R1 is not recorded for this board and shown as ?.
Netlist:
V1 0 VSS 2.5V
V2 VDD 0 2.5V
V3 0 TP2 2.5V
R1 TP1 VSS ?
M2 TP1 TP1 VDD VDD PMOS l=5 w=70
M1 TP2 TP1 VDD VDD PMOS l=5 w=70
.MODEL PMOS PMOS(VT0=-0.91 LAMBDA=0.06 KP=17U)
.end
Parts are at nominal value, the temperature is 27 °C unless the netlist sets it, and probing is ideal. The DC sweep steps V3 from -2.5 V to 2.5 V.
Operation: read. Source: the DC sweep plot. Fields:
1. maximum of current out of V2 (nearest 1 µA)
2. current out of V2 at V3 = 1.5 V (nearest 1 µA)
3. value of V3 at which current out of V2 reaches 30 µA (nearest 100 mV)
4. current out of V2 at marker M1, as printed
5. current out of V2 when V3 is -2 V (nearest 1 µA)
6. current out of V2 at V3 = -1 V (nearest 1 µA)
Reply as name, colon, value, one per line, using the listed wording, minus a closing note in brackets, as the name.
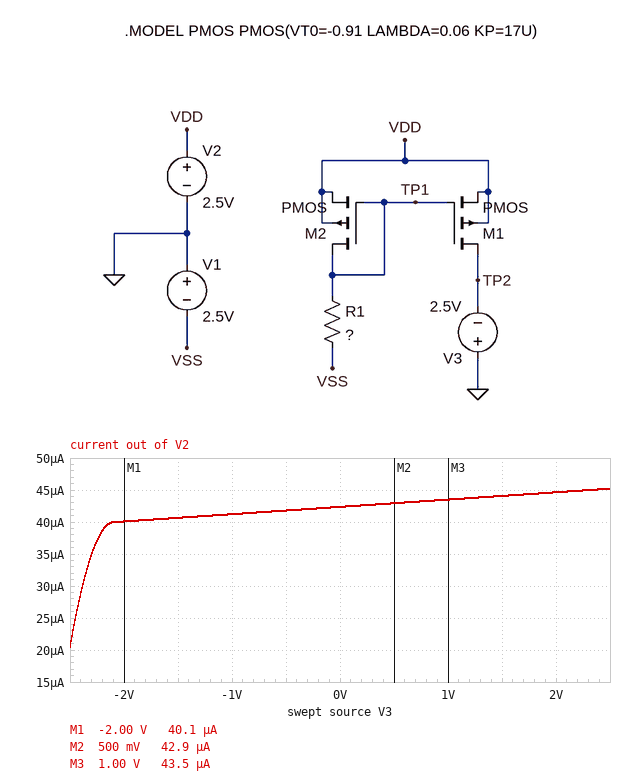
maximum of current out of V2: 45 µA
current out of V2 at V3 = 1.5 V: 44 µA
value of V3 at which current out of V2 reaches 30 µA: -2.4 V
current out of V2 at marker M1, as printed: 40.1 µA
current out of V2 when V3 is -2 V: 40 µA
current out of V2 at V3 = -1 V: 41 µA
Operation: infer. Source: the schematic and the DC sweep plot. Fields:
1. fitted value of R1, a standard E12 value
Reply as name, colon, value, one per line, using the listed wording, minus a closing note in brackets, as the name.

fitted value of R1, a standard E12 value: 180 kΩ
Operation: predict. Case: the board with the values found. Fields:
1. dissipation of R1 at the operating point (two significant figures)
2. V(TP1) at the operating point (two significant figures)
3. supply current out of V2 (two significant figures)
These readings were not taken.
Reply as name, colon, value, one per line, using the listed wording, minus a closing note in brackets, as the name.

dissipation of R1 at the operating point: 76 µW
V(TP1) at the operating point: 1.2 V
supply current out of V2: 45 µA
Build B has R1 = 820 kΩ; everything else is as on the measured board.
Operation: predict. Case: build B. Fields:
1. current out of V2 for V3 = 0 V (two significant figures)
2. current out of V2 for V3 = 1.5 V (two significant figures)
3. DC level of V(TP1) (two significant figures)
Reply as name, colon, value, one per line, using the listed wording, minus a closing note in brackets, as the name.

current out of V2 for V3 = 0 V: 9.9 µA
current out of V2 for V3 = 1.5 V: 10 µA
DC level of V(TP1): 1.4 V
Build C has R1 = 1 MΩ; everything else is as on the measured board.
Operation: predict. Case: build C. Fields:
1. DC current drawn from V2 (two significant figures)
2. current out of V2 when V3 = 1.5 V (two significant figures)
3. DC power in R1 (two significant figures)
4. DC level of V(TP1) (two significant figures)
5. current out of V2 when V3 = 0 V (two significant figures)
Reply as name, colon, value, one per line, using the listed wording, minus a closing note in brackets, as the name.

DC current drawn from V2: 8.7 µA
current out of V2 when V3 = 1.5 V: 8.5 µA
DC power in R1: 15 µW
DC level of V(TP1): 1.4 V
current out of V2 when V3 = 0 V: 8.1 µA
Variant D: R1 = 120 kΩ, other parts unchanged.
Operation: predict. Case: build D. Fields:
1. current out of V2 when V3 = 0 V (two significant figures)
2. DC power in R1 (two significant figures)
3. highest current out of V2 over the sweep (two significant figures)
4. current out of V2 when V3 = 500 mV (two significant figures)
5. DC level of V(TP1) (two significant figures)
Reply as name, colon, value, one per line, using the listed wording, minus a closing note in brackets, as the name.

current out of V2 when V3 = 0 V: 62 µA
DC power in R1: 110 µW
highest current out of V2 over the sweep: 66 µA
current out of V2 when V3 = 500 mV: 63 µA
DC level of V(TP1): 1.1 V
